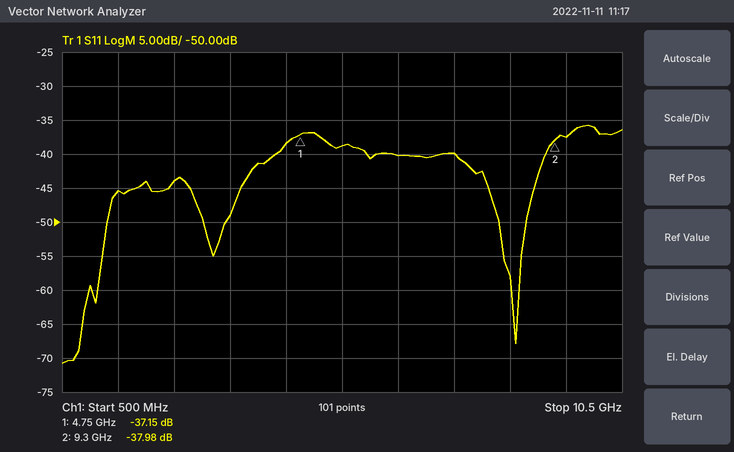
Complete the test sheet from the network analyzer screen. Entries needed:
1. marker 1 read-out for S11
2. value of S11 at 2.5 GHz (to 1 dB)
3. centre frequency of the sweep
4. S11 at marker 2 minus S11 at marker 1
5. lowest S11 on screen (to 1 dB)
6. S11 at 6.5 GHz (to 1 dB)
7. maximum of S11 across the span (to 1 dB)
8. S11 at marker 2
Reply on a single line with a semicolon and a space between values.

-37.15 dB; -44 dB; 5.5 GHz; -0.83 dB; -71 dB; -40 dB; -36 dB; -37.98 dB
